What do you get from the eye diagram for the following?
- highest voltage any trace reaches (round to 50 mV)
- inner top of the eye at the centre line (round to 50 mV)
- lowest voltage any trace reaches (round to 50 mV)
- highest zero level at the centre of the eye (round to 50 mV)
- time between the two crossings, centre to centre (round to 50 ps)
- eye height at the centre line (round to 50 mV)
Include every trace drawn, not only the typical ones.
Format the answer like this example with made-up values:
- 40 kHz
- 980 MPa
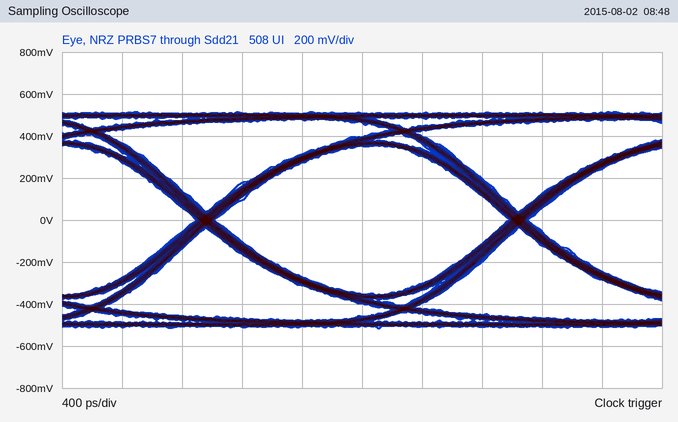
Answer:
- 500 mV
- 350 mV
- -500 mV
- -350 mV
- 2.10 ns
- 700 mV
